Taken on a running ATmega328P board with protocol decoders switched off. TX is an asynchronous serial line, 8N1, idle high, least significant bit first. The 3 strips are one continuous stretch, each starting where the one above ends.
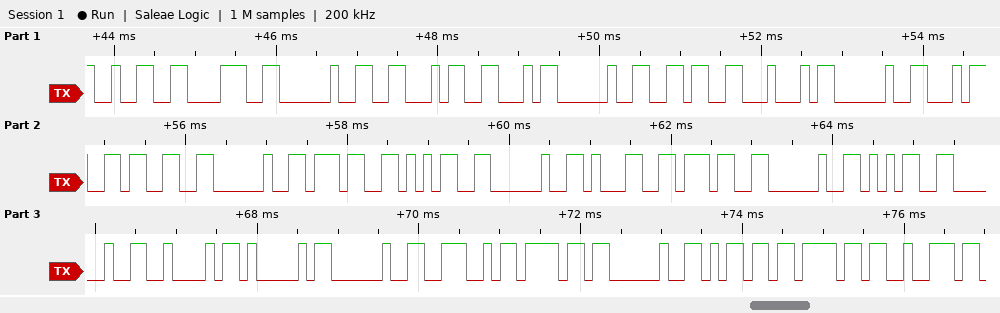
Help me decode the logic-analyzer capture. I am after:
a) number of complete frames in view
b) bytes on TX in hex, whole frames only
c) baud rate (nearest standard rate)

29
32 38 20 46 46 20 36 44 20 34 33 20 37 35 20 31 37 20 35 20 42 41 20 4E 6F 20 6D 6F 72
9600 baud
